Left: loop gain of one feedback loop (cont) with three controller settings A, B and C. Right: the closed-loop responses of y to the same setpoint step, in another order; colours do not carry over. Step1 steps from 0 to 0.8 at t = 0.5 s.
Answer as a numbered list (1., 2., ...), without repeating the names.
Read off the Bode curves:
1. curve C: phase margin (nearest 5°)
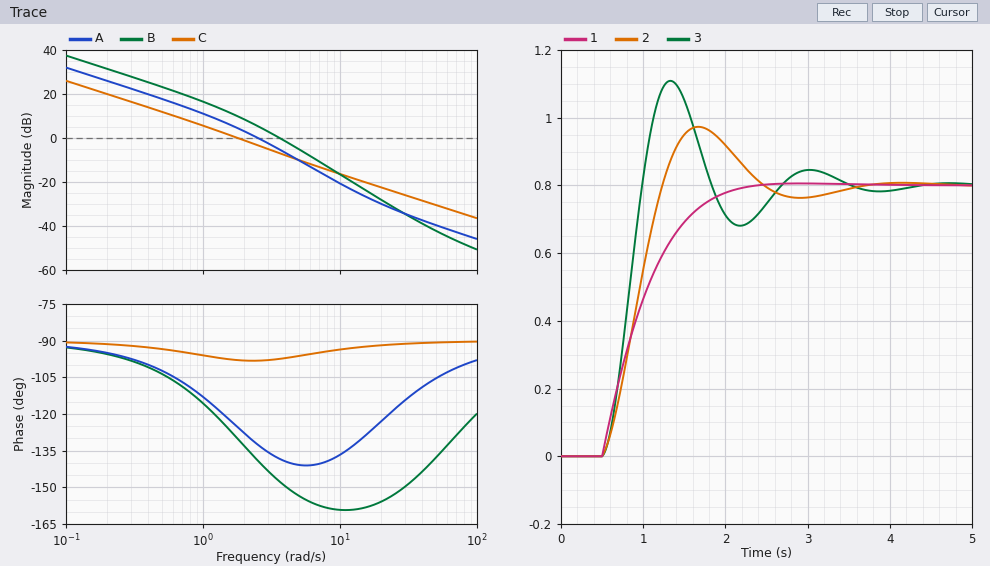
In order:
1. 80°
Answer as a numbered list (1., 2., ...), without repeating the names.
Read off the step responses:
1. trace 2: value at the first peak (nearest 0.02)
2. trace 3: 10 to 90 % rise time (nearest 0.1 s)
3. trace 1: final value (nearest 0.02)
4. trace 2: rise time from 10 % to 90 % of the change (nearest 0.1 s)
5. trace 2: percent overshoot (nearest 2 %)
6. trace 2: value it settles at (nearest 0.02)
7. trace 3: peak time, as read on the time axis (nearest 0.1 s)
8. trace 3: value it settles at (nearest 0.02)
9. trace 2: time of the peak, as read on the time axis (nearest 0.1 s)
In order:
1. 0.98
2. 0.3 s
3. 0.80
4. 0.5 s
5. 22 %
6. 0.80
7. 1.3 s
8. 0.80
9. 1.7 s
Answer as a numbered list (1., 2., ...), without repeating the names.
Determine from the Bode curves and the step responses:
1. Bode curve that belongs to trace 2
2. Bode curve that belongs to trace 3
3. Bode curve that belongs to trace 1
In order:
1. A
2. B
3. C
